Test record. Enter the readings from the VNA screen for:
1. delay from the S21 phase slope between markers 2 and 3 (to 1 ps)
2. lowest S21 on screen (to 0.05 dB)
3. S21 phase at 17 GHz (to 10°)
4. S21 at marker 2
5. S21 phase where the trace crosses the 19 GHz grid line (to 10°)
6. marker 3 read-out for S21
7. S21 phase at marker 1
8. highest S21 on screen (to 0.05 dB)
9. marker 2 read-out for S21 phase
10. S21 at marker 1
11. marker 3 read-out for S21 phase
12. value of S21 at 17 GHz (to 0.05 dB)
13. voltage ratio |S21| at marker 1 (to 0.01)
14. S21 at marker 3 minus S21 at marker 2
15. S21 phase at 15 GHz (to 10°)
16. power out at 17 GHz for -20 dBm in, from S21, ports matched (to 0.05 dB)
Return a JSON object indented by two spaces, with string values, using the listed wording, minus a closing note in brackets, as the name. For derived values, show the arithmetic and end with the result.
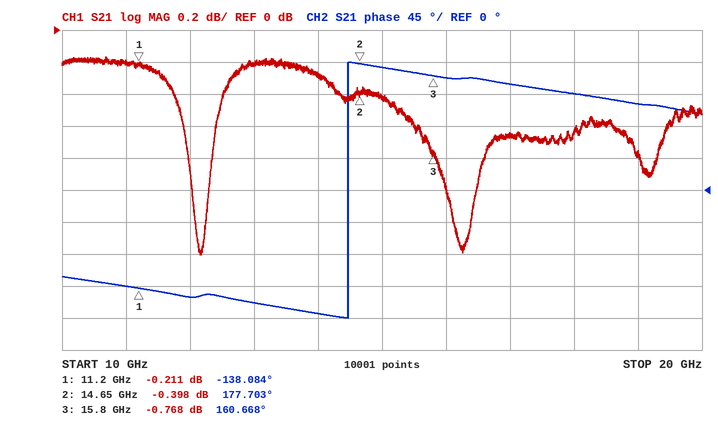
{
  "delay from the S21 phase slope between markers 2 and 3": "−(160.668° − (177.703°))/(360° × 1.15 GHz) ≈ 41 ps",
  "lowest S21 on screen": "-1.40 dB",
  "S21 phase at 17 GHz": "150°",
  "S21 at marker 2": "-0.398 dB",
  "S21 phase where the trace crosses the 19 GHz grid line": "120°",
  "marker 3 read-out for S21": "-0.768 dB",
  "S21 phase at marker 1": "-138.084°",
  "highest S21 on screen": "-0.15 dB",
  "marker 2 read-out for S21 phase": "177.703°",
  "S21 at marker 1": "-0.211 dB",
  "marker 3 read-out for S21 phase": "160.668°",
  "value of S21 at 17 GHz": "-0.65 dB",
  "voltage ratio |S21| at marker 1": "10^(-0.211/20) ≈ 0.98",
  "S21 at marker 3 minus S21 at marker 2": "-0.768 − (-0.398) = -0.370 dB",
  "S21 phase at 15 GHz": "170°",
  "power out at 17 GHz for -20 dBm in, from S21, ports matched": "-20 dBm + (-0.65 dB) = -20.65 dBm"
}
